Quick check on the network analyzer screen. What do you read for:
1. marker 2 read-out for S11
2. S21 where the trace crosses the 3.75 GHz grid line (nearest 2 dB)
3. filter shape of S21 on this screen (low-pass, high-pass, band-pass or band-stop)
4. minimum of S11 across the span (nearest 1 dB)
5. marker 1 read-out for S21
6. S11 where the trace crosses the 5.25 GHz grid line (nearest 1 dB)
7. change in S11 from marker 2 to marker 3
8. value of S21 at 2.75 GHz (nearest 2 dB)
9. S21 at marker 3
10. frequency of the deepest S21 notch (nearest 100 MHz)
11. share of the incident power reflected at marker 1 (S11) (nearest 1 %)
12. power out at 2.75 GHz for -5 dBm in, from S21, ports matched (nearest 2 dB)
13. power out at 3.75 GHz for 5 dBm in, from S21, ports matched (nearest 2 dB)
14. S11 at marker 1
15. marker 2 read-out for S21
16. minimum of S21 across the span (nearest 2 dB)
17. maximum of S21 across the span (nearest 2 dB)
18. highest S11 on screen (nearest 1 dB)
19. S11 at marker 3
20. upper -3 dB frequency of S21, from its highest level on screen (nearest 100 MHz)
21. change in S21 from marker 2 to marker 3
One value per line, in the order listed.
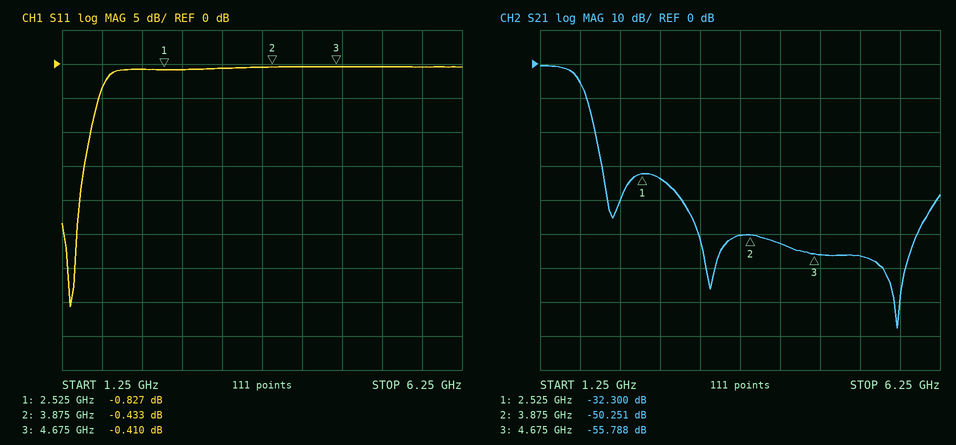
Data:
-0.433 dB
-50 dB
low-pass
-36 dB
-32.300 dB
0 dB
0.023 dB
-34 dB
-55.788 dB
5.7 GHz
83 %
-38 dBm
-46 dBm
-0.827 dB
-50.251 dB
-78 dB
0 dB
0 dB
-0.410 dB
1.7 GHz
-5.537 dB
